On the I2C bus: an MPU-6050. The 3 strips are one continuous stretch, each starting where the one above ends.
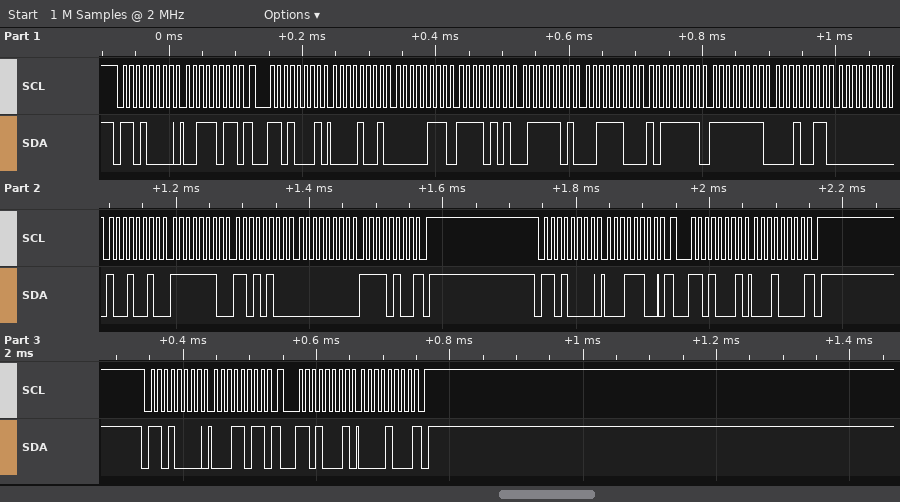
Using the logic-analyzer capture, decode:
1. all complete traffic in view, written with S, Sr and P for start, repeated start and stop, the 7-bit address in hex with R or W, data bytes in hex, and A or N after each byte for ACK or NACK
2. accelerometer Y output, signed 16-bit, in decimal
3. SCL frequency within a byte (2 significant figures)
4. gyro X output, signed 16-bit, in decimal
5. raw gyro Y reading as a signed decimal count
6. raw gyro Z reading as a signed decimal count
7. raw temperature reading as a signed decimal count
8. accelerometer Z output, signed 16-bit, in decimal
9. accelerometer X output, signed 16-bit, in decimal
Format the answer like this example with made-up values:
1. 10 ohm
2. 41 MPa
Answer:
1. S 68W A 3B A Sr 68R A 09 A 07 A F5 A 7D A 3C A BF A FF A 13 A 00 A 92 A FE A D4 A 00 A F4 N P S 68W A 1C A Sr 68R A 10 N P S 68W A 1B A Sr 68R A 08 N P
2. -2691
3. 100 kHz
4. 146
5. -300
6. 244
7. -237
8. 15551
9. 2311
